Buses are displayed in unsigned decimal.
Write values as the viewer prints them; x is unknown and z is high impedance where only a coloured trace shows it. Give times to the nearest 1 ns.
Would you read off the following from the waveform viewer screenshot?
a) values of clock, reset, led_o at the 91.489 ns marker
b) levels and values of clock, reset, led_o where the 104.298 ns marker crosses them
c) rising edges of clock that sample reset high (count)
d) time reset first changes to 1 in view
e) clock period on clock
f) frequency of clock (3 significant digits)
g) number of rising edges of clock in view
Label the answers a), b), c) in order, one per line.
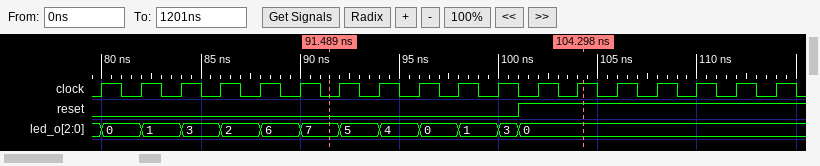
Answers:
a) clock=0, reset=0, led_o=7
b) clock=1, reset=1, led_o=0
c) 7
d) 101 ns
e) 2 ns
f) 500 MHz
g) 18
